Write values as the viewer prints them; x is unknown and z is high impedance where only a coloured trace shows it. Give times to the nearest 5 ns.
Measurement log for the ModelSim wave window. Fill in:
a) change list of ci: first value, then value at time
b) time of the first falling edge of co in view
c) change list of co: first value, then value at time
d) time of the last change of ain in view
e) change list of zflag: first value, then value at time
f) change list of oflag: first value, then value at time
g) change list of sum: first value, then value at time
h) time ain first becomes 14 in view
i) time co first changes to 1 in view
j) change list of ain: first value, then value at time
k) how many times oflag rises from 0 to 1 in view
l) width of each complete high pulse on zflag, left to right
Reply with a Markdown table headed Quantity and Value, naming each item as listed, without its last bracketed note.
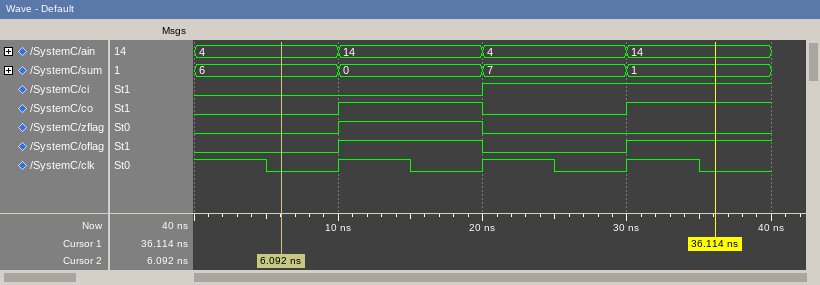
| Quantity | Value |
|---|---|
| change list of ci: first value, then value at time | 0, 1 at 20 ns |
| time of the first falling edge of co in view | 20 ns |
| change list of co: first value, then value at time | 0, 1 at 10 ns, 0 at 20 ns, 1 at 30 ns |
| time of the last change of ain in view | 30 ns |
| change list of zflag: first value, then value at time | 0, 1 at 10 ns, 0 at 20 ns |
| change list of oflag: first value, then value at time | 0, 1 at 10 ns, 0 at 20 ns, 1 at 30 ns |
| change list of sum: first value, then value at time | 6, 0 at 10 ns, 7 at 20 ns, 1 at 30 ns |
| time ain first becomes 14 in view | 10 ns |
| time co first changes to 1 in view | 10 ns |
| change list of ain: first value, then value at time | 4, 14 at 10 ns, 4 at 20 ns, 14 at 30 ns |
| how many times oflag rises from 0 to 1 in view | 2 |
| width of each complete high pulse on zflag, left to right | 10 ns |
